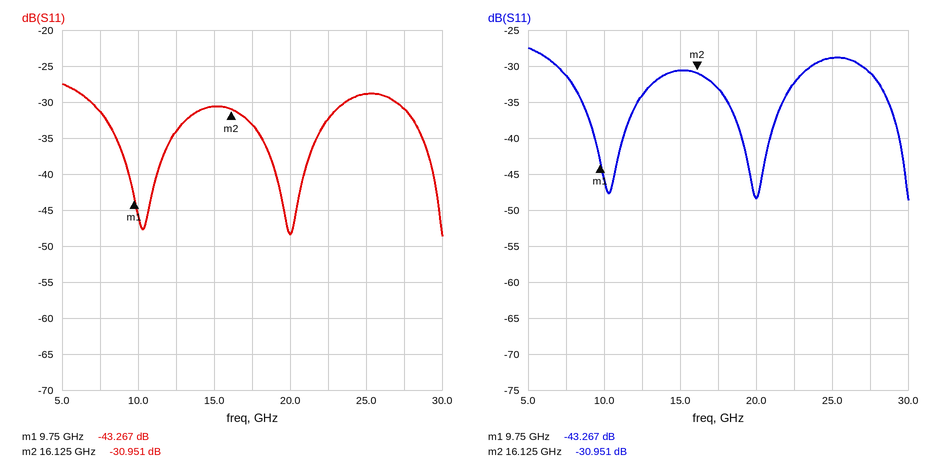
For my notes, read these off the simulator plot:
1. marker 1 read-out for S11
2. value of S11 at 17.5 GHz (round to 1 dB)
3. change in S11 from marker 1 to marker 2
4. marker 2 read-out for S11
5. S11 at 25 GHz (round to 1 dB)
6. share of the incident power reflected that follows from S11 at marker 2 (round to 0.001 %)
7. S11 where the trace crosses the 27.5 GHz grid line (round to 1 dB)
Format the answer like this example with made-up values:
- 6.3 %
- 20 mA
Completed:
- -43.267 dB
- -33 dB
- 12.316 dB
- -30.951 dB
- -29 dB
- 0.080 %
- -31 dB
